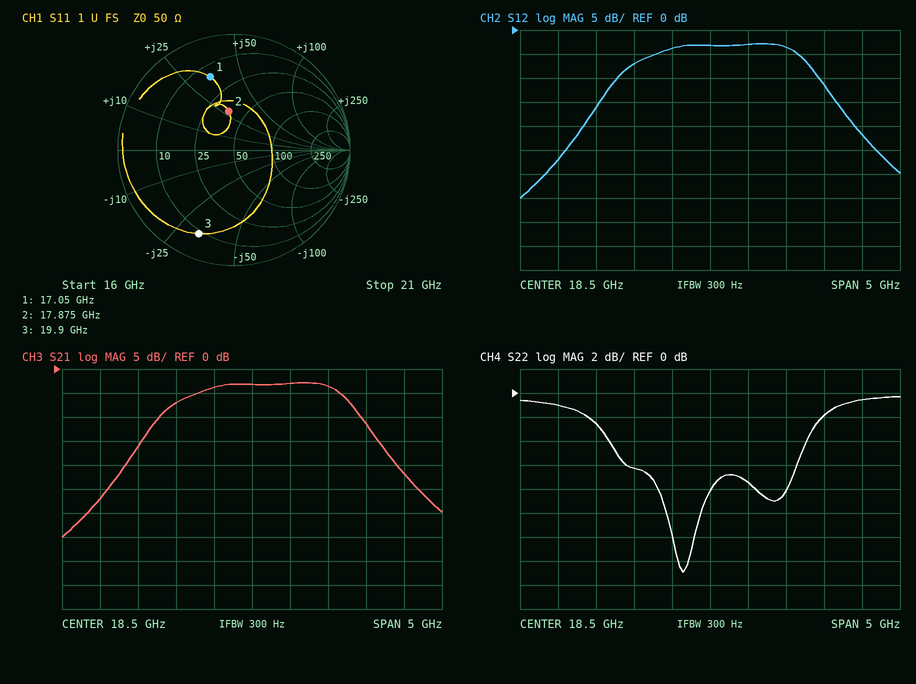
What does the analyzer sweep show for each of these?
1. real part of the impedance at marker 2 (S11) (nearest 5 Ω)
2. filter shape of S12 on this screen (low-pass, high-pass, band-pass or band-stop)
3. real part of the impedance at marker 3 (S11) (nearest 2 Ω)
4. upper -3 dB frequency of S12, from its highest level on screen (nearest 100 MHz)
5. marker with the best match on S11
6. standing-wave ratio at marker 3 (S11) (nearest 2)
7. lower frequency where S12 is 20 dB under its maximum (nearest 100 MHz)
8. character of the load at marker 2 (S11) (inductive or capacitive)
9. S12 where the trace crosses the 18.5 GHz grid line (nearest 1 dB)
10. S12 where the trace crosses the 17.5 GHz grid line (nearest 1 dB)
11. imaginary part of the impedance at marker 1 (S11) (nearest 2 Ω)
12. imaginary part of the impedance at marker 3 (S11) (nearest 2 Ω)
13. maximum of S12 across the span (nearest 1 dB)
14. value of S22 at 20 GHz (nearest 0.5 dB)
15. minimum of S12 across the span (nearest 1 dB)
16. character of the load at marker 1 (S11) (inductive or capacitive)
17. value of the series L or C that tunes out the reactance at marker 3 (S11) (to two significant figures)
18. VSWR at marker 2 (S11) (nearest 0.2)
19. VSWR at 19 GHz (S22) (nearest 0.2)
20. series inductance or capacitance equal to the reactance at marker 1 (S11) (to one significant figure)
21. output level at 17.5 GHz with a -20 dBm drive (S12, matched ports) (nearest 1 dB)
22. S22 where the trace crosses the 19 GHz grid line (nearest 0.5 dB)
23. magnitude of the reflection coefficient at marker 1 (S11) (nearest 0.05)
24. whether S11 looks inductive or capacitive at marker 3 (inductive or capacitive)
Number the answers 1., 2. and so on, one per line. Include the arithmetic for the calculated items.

1. 35 Ω
2. band-pass
3. 8 Ω
4. 19.7 GHz
5. marker 2
6. 8
7. 16.7 GHz
8. inductive
9. -3 dB
10. -7 dB
11. +34 Ω
12. -32 Ω
13. -3 dB
14. -2.0 dB
15. -35 dB
16. inductive
17. L = 32 Ω/(2π × 19.9 GHz) ≈ 256 pH, so 260 pH to two significant figures
18. 2.0
19. |Γ| = 10^(-7.5/20) = 0.4217; VSWR = (1 + 0.4217)/(1 − 0.4217) ≈ 2.46, so 2.4 to the nearest 0.2
20. L = 34 Ω/(2π × 17.05 GHz) ≈ 317 pH, so 300 pH to one significant figure
21. -20 dBm + (-7 dB) = -27 dBm
22. -7.5 dB
23. 0.65
24. capacitive
